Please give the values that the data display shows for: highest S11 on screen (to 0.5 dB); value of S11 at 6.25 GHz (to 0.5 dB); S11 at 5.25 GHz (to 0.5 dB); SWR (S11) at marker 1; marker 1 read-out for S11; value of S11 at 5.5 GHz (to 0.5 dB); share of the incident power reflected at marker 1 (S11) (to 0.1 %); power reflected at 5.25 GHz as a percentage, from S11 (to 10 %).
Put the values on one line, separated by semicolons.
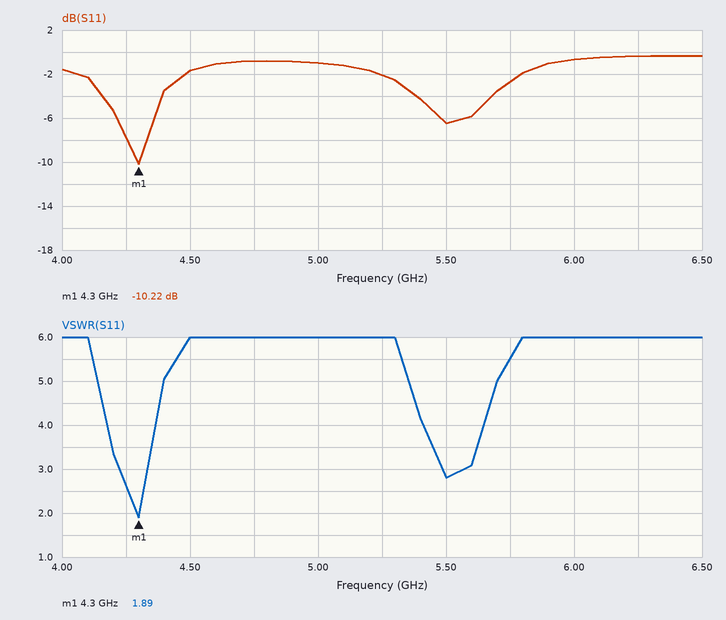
-0.5 dB; -0.5 dB; -2.0 dB; 1.89; -10.22 dB; -6.5 dB; 9.5 %; 60 %
